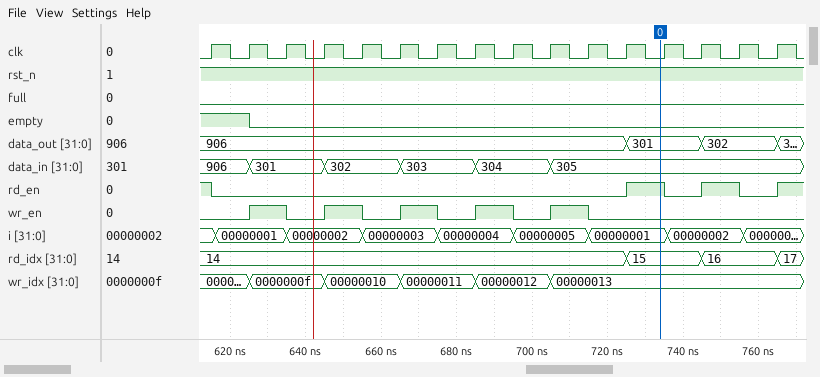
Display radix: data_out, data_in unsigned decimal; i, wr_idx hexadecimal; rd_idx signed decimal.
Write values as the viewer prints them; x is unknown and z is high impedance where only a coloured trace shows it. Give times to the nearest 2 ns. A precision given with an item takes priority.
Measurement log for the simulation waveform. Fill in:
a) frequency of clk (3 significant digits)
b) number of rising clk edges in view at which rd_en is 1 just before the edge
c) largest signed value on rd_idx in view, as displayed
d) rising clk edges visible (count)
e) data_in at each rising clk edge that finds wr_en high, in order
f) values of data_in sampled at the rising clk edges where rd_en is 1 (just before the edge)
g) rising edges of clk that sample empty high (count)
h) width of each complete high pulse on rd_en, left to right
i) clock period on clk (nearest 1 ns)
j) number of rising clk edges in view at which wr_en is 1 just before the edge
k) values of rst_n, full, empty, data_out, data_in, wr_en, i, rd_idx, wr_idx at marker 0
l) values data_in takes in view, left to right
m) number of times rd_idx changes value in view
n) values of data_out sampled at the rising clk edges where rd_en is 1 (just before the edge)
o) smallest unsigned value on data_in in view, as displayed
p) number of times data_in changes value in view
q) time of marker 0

100 MHz
3
17
16
301, 302, 303, 304, 305
906, 305, 305
2
10 ns, 10 ns
10 ns
5
rst_n=1, full=0, empty=0, data_out=301, data_in=305, wr_en=0, i=00000001, rd_idx=15, wr_idx=00000013
906, 301, 302, 303, 304, 305
3
906, 301, 302
301
5
734 ns
